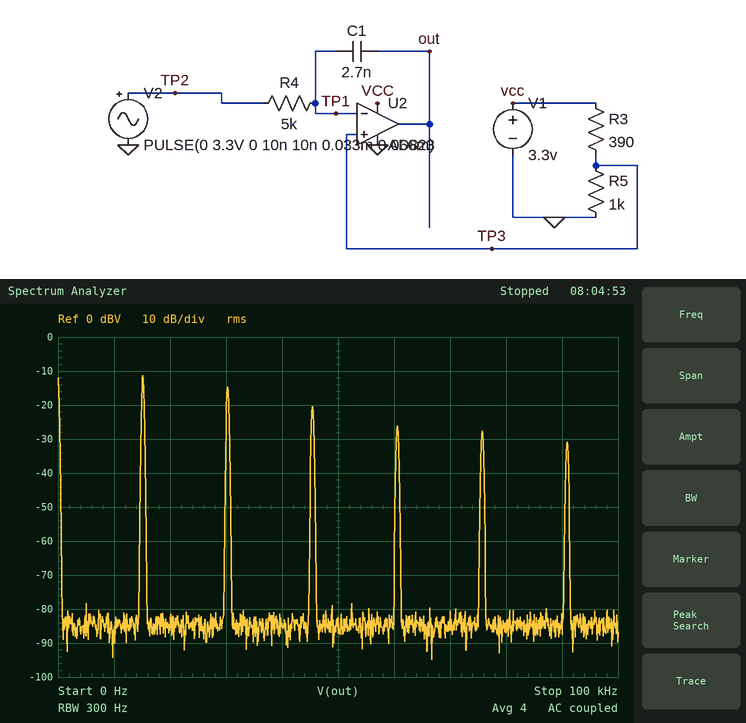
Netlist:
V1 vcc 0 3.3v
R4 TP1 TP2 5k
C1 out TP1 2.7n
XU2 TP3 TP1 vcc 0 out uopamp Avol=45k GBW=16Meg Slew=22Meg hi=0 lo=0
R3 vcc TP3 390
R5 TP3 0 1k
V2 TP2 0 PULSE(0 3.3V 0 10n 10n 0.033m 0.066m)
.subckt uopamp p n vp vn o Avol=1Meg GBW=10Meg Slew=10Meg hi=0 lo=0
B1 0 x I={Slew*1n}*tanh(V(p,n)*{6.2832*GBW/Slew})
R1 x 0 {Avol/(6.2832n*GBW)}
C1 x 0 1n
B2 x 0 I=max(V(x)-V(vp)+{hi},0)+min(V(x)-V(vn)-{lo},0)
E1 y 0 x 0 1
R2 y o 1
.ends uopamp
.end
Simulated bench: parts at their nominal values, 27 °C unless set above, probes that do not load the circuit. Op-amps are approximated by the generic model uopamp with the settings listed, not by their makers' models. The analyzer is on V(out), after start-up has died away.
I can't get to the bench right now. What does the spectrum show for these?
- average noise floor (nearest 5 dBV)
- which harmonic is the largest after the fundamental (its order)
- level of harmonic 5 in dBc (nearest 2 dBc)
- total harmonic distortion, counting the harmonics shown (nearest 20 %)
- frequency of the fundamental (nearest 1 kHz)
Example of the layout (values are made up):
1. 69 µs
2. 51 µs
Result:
1. -85 dBV
2. 2
3. -16 dBc
4. 80 %
5. 15 kHz
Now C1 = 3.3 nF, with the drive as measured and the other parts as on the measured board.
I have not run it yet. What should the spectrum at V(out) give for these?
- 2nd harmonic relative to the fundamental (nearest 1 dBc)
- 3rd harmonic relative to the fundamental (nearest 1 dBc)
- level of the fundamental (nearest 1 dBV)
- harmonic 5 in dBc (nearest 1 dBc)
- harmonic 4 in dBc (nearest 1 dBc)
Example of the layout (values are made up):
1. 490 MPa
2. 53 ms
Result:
1. -2 dBc
2. -6 dBc
3. -16 dBV
4. -16 dBc
5. -12 dBc
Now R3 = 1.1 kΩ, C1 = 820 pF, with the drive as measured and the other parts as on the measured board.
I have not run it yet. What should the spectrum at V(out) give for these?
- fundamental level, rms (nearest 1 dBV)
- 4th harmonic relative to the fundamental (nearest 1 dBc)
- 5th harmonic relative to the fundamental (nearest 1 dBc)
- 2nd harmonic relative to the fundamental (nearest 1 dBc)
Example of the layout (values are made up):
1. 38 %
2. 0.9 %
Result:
1. 3 dBV
2. -32 dBc
3. -21 dBc
4. -29 dBc
